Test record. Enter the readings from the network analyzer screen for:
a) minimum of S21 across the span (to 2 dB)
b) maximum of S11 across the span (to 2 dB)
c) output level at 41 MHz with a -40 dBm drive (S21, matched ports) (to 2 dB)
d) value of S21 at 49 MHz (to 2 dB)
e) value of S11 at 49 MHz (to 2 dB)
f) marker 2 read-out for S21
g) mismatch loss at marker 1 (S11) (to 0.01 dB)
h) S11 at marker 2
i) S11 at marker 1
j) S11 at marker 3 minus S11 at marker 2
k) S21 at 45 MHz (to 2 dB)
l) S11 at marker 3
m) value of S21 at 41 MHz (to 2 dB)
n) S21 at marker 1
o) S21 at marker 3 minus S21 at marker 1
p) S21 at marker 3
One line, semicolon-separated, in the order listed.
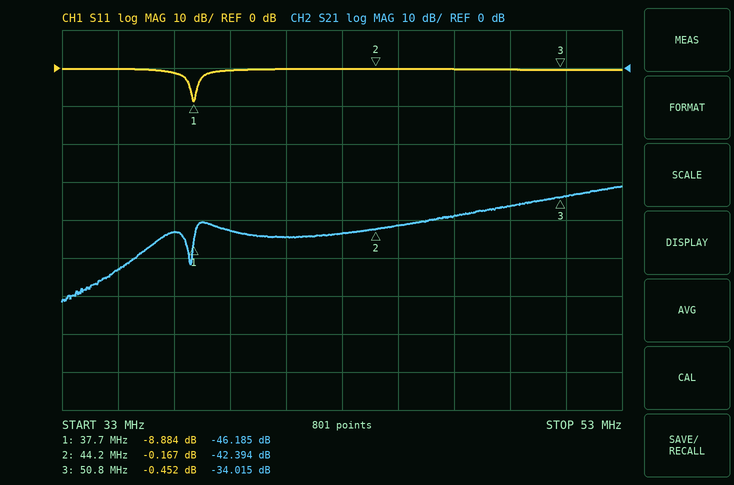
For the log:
-62 dB; 0 dB; -84 dBm; -36 dB; 0 dB; -42.394 dB; 0.60 dB; -0.167 dB; -8.884 dB; -0.285 dB; -42 dB; -0.452 dB; -44 dB; -46.185 dB; 12.170 dB; -34.015 dB
